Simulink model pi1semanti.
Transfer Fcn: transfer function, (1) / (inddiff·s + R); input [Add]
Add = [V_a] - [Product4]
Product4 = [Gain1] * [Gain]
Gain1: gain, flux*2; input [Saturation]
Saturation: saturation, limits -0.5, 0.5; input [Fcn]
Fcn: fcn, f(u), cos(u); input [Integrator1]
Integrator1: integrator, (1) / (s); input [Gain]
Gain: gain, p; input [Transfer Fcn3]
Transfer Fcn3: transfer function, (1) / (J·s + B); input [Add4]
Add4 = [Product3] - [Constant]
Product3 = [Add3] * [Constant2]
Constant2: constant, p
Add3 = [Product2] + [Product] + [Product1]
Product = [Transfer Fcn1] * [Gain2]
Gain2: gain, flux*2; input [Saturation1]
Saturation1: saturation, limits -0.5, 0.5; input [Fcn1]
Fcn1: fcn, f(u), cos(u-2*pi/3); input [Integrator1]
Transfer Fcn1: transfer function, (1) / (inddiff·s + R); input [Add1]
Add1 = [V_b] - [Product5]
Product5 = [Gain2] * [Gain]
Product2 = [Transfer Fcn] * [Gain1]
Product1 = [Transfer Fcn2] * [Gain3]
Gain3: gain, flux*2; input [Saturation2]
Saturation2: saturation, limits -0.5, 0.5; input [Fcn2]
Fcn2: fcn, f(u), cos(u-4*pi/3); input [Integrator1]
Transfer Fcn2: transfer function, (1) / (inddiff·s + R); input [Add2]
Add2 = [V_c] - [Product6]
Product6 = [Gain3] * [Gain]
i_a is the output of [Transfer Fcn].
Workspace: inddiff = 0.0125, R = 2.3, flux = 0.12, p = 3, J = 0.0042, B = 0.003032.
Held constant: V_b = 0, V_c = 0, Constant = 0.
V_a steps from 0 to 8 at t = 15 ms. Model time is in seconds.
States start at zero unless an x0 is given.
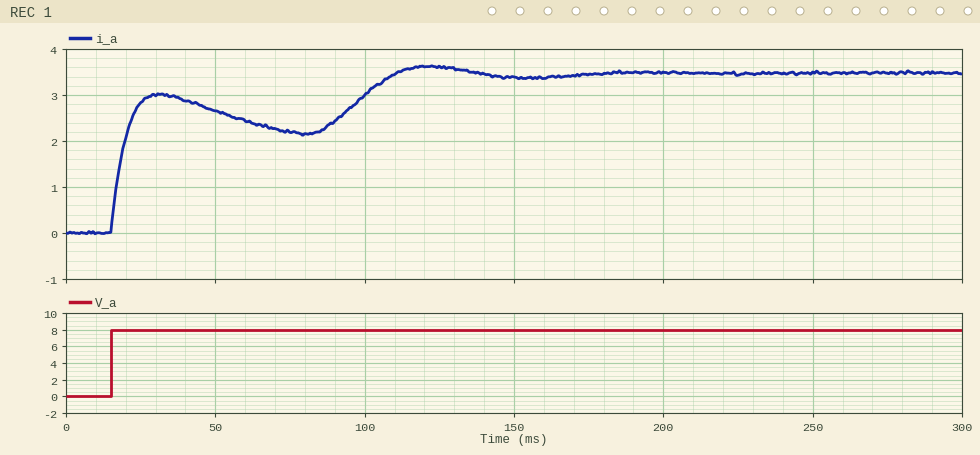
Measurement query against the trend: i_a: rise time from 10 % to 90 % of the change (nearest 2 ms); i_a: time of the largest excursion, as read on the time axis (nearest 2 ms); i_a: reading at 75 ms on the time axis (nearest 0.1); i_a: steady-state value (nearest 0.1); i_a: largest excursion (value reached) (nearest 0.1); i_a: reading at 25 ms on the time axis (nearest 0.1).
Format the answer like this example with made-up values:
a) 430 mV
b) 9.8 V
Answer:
a) 86 ms
b) 122 ms
c) 2.2
d) 3.5
e) 3.6
f) 2.8
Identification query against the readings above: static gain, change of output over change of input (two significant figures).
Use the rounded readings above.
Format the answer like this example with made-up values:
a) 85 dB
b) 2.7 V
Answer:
a) 0.44
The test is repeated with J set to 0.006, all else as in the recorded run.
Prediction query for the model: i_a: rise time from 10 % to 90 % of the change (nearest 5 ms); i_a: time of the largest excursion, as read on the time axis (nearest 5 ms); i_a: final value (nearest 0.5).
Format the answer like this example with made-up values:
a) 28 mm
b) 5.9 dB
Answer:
a) 95 ms
b) 135 ms
c) 3.5
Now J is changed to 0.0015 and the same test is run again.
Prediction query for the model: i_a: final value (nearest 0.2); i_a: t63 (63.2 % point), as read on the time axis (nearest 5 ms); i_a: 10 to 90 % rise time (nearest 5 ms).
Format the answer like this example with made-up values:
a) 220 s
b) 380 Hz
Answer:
a) 3.4
b) 20 ms
c) 70 ms
